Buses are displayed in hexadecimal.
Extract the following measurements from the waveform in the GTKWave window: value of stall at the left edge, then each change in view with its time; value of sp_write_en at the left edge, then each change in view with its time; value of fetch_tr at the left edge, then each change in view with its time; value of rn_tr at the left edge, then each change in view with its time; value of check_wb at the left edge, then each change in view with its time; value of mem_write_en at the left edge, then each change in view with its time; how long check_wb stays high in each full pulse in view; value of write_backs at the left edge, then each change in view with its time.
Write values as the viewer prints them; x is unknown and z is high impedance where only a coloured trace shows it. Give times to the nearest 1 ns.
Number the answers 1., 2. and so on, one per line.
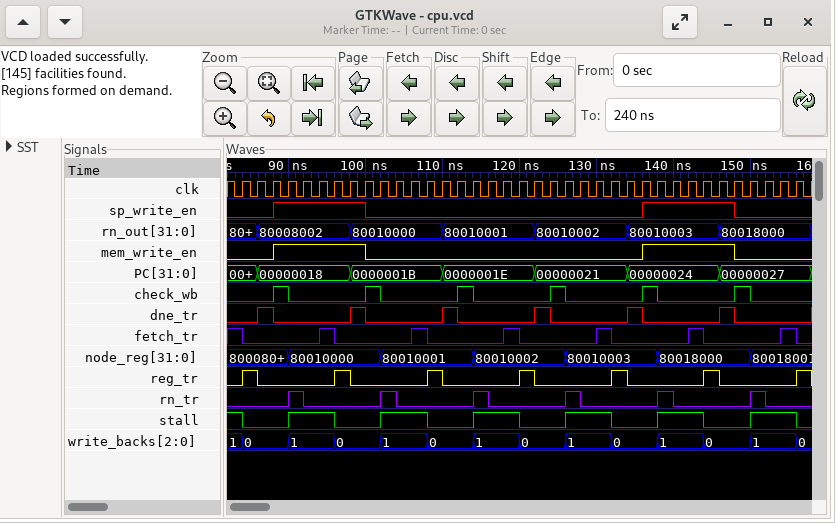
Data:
1. 1, 0 at 84 ns, 1 at 90 ns, 0 at 96 ns, 1 at 102 ns, 0 at 108 ns, 1 at 114 ns, 0 at 120 ns, 1 at 126 ns, 0 at 132 ns, 1 at 138 ns, 0 at 144 ns, 1 at 150 ns, 0 at 156 ns
2. 0, 1 at 88 ns, 0 at 100 ns, 1 at 136 ns, 0 at 148 ns
3. 1, 0 at 84 ns, 1 at 94 ns, 0 at 96 ns, 1 at 106 ns, 0 at 108 ns, 1 at 118 ns, 0 at 120 ns, 1 at 130 ns, 0 at 132 ns, 1 at 142 ns, 0 at 144 ns, 1 at 154 ns, 0 at 156 ns
4. 0, 1 at 90 ns, 0 at 92 ns, 1 at 102 ns, 0 at 104 ns, 1 at 114 ns, 0 at 116 ns, 1 at 126 ns, 0 at 128 ns, 1 at 138 ns, 0 at 140 ns, 1 at 150 ns, 0 at 152 ns
5. 0, 1 at 88 ns, 0 at 90 ns, 1 at 100 ns, 0 at 102 ns, 1 at 112 ns, 0 at 114 ns, 1 at 124 ns, 0 at 126 ns, 1 at 136 ns, 0 at 138 ns, 1 at 148 ns, 0 at 150 ns
6. 0, 1 at 88 ns, 0 at 100 ns, 1 at 136 ns, 0 at 148 ns
7. 2 ns, 2 ns, 2 ns, 2 ns, 2 ns, 2 ns
8. 1, 0 at 84 ns, 1 at 90 ns, 0 at 96 ns, 1 at 102 ns, 0 at 108 ns, 1 at 114 ns, 0 at 120 ns, 1 at 126 ns, 0 at 132 ns, 1 at 138 ns, 0 at 144 ns, 1 at 150 ns, 0 at 156 ns
